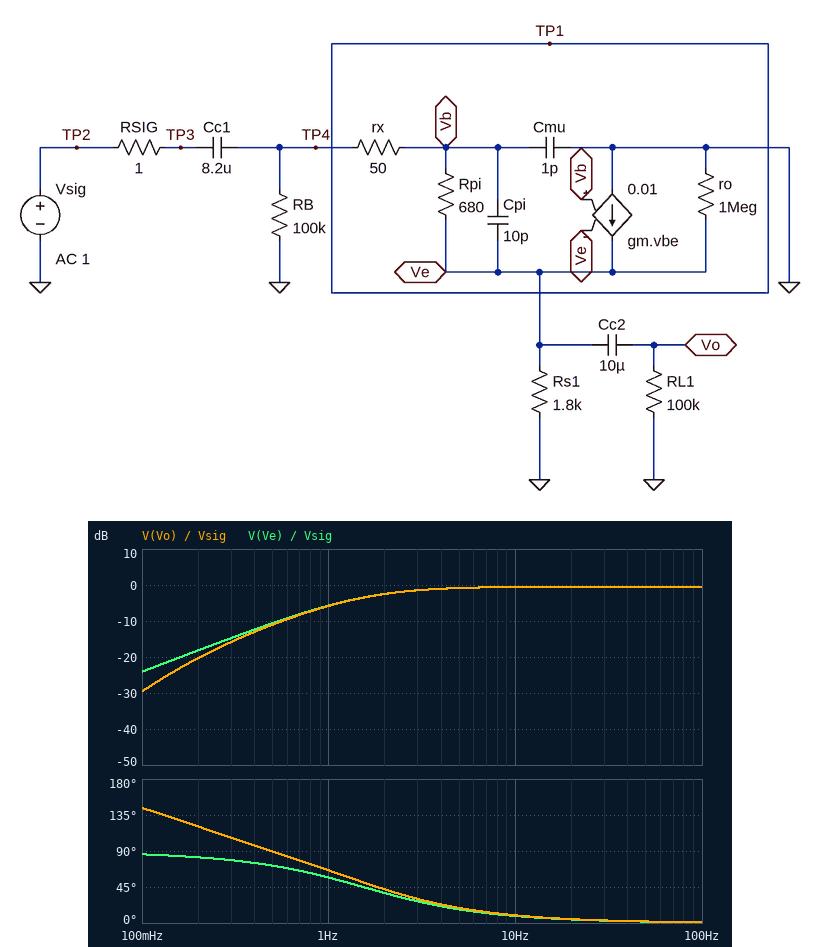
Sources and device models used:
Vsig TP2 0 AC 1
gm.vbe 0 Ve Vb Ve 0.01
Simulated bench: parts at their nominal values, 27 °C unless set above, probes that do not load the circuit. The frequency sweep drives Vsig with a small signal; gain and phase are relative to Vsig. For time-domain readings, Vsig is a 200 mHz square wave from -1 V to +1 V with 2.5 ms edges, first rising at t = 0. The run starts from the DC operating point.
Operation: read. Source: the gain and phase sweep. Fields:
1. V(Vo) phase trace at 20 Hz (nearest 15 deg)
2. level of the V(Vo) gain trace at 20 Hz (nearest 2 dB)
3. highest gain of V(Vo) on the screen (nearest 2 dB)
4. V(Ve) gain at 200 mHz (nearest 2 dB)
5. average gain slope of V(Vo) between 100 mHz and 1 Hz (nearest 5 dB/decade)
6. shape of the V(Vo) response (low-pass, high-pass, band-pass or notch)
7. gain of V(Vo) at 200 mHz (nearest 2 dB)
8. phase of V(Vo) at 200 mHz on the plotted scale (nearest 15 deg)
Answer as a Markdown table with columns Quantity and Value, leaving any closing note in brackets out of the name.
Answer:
| Quantity | Value |
|---|---|
| V(Vo) phase trace at 20 Hz | 0 deg |
| level of the V(Vo) gain trace at 20 Hz | 0 dB |
| highest gain of V(Vo) on the screen | 0 dB |
| V(Ve) gain at 200 mHz | -18 dB |
| average gain slope of V(Vo) between 100 mHz and 1 Hz | 25 dB/decade |
| shape of the V(Vo) response | high-pass |
| gain of V(Vo) at 200 mHz | -20 dB |
| phase of V(Vo) at 200 mHz on the plotted scale | 120 deg |
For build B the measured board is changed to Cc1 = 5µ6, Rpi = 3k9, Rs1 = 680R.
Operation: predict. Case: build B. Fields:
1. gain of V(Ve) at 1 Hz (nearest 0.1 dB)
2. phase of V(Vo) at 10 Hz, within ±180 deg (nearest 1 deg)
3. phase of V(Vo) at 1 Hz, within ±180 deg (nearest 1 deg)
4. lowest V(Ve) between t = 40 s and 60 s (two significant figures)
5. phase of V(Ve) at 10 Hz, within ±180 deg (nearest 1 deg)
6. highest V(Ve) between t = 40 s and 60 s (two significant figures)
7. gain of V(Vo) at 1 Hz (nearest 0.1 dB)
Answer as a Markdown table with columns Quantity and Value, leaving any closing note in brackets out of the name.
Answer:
| Quantity | Value |
|---|---|
| gain of V(Ve) at 1 Hz | -5.1 dB |
| phase of V(Vo) at 10 Hz, within ±180 deg | 8 deg |
| phase of V(Vo) at 1 Hz, within ±180 deg | 59 deg |
| lowest V(Ve) between t = 40 s and 60 s | -1.7 V |
| phase of V(Ve) at 10 Hz, within ±180 deg | 7 deg |
| highest V(Ve) between t = 40 s and 60 s | 1.7 V |
| gain of V(Vo) at 1 Hz | -5.2 dB |
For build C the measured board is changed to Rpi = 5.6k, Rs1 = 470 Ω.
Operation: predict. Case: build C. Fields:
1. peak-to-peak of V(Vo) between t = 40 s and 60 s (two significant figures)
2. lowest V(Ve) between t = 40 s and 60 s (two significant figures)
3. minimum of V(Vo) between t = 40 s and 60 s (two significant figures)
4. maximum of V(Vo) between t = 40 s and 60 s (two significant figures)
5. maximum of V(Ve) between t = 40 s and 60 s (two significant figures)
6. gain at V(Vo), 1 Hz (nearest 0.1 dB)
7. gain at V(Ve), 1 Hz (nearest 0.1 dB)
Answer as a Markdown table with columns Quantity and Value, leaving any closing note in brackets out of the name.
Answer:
| Quantity | Value |
|---|---|
| peak-to-peak of V(Vo) between t = 40 s and 60 s | 3.3 V |
| lowest V(Ve) between t = 40 s and 60 s | -1.6 V |
| minimum of V(Vo) between t = 40 s and 60 s | -1.7 V |
| maximum of V(Vo) between t = 40 s and 60 s | 1.7 V |
| maximum of V(Ve) between t = 40 s and 60 s | 1.6 V |
| gain at V(Vo), 1 Hz | -3.9 dB |
| gain at V(Ve), 1 Hz | -3.8 dB |
